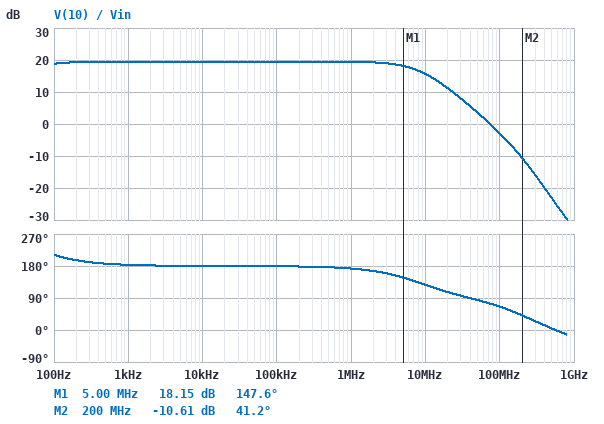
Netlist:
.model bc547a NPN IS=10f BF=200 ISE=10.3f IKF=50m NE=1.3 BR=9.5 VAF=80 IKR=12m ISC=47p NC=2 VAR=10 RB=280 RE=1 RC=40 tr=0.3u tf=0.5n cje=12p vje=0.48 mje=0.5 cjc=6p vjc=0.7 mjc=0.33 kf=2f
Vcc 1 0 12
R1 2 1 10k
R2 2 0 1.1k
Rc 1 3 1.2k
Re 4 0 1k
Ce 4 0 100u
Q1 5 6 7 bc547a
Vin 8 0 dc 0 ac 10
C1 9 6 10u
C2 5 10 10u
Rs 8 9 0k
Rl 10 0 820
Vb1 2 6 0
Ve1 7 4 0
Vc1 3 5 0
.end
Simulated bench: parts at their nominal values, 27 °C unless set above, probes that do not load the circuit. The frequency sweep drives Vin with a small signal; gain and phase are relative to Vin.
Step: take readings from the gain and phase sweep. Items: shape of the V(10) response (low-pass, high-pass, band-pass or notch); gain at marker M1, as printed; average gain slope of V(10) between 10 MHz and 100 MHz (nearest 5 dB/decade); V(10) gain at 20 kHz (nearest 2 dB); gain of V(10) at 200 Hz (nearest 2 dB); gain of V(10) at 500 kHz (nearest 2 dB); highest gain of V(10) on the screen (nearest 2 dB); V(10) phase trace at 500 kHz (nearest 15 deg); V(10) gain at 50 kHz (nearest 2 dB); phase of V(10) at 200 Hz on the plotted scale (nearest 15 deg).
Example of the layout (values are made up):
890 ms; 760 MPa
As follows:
low-pass; 18.15 dB; -20 dB/decade; 20 dB; 20 dB; 20 dB; 20 dB; 180 deg; 20 dB; 195 deg
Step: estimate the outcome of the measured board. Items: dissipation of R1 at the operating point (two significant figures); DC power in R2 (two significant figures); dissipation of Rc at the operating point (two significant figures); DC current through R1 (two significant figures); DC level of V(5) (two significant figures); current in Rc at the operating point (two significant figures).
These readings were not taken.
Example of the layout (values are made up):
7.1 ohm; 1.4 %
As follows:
12 mW; 1.3 mW; 350 µW; 1.1 mA; 11 V; 540 µA
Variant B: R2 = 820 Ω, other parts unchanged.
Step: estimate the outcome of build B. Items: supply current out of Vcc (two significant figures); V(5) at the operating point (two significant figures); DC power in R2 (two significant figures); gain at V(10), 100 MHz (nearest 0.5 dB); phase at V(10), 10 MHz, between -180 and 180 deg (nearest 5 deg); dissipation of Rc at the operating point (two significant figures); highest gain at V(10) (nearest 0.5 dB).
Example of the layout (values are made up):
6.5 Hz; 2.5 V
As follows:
1.4 mA; 12 V; 1.0 mW; -6.0 dB; 135 deg; 96 µW; 14.0 dB
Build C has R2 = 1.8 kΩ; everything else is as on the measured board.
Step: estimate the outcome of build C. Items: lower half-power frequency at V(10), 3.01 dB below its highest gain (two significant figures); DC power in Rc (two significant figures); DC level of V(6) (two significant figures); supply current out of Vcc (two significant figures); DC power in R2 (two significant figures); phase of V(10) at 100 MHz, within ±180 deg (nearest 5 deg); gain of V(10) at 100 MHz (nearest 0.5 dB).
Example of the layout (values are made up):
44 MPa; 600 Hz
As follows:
70 Hz; 1.6 mW; 1.8 V; 2.2 mA; 1.8 mW; 70 deg; -0.5 dB
